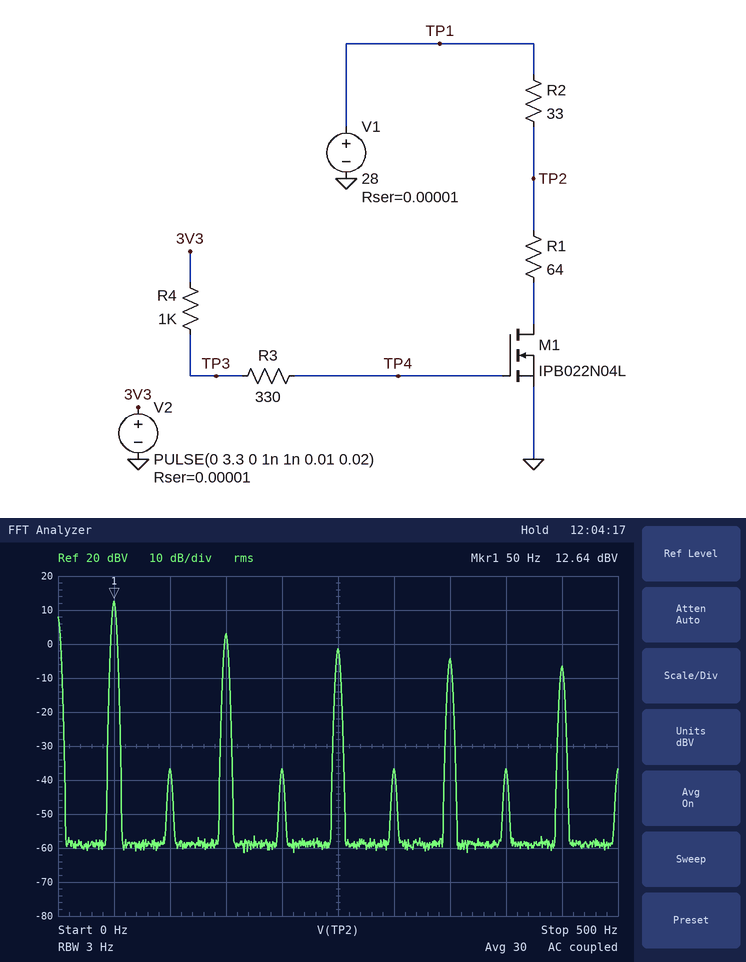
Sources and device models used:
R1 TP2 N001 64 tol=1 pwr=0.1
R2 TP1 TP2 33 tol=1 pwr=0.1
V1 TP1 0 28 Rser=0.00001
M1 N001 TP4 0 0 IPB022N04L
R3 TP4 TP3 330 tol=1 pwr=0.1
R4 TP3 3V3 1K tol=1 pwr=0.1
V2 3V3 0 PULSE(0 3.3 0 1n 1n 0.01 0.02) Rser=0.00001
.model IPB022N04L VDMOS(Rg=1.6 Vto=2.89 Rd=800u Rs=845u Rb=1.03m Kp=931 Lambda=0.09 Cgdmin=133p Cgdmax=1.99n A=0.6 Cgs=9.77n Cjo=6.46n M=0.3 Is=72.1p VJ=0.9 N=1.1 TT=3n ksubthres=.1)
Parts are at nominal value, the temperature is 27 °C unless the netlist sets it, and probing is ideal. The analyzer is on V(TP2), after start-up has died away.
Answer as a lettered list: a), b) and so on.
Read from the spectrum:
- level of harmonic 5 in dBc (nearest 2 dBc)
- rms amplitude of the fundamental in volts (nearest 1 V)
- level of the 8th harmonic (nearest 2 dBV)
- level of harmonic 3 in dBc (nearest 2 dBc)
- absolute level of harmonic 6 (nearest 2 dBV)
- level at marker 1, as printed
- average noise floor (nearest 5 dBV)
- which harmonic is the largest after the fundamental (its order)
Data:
a) -14 dBc
b) 4 V
c) -36 dBV
d) -10 dBc
e) -36 dBV
f) 12.64 dBV
g) -60 dBV
h) 3
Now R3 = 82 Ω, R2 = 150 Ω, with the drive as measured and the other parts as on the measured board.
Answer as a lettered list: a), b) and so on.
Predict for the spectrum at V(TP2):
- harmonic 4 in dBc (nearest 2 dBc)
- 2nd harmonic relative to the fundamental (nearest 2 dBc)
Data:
a) -52 dBc
b) -52 dBc
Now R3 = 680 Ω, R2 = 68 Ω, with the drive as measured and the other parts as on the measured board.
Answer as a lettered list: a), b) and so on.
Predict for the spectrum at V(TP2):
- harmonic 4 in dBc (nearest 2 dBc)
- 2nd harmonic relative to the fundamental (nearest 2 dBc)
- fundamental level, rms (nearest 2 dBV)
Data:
a) -48 dBc
b) -48 dBc
c) 16 dBV
